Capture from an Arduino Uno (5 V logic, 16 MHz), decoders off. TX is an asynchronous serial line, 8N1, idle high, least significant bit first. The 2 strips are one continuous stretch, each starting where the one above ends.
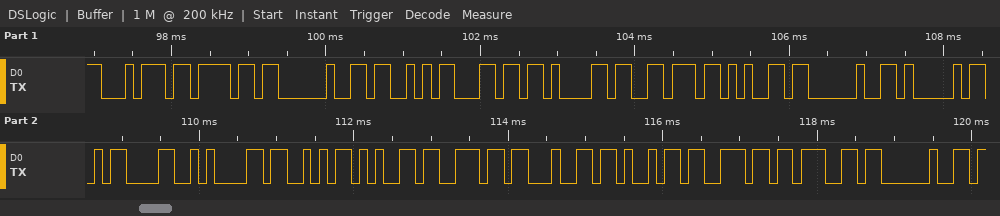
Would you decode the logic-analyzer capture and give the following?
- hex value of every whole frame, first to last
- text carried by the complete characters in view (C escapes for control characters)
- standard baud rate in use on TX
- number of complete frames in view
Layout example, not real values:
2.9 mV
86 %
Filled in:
74 6F 20 53 6C 61 76 65 20 41 0D 0A 53 65 6E 64 69 6E 67 20
"to Slave A\r\nSending "
9600 baud
20
